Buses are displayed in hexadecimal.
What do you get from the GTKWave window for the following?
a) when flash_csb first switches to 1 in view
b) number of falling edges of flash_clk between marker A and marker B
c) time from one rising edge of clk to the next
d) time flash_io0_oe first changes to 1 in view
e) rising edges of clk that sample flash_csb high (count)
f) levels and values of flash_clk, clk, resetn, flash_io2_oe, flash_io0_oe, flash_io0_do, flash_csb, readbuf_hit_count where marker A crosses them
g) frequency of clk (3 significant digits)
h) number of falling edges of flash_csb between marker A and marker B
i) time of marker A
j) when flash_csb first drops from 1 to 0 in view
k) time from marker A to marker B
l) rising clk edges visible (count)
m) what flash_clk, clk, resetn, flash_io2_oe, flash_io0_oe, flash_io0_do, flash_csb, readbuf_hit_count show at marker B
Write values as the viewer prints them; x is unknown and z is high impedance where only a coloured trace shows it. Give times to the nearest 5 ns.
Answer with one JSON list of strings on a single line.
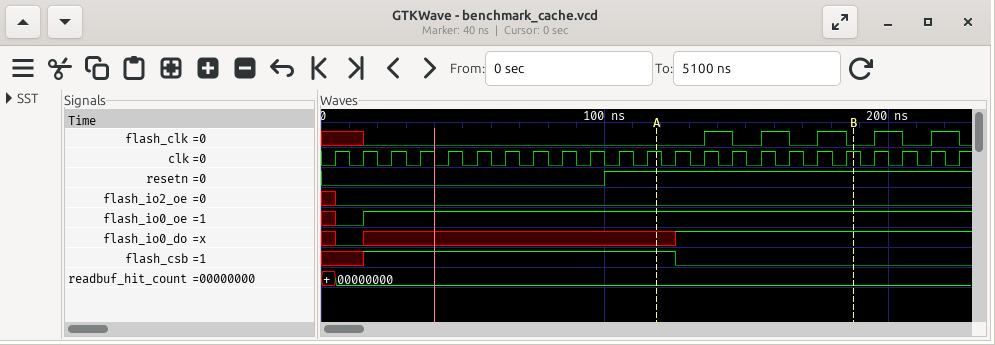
["15 ns", "3", "10 ns", "15 ns", "11", "flash_clk=0, clk=1, resetn=1, flash_io2_oe=0, flash_io0_oe=1, flash_io0_do=x, flash_csb=1, readbuf_hit_count=00000000", "100 MHz", "1", "120 ns", "125 ns", "70 ns", "23", "flash_clk=0, clk=1, resetn=1, flash_io2_oe=0, flash_io0_oe=1, flash_io0_do=1, flash_csb=0, readbuf_hit_count=00000000"]
